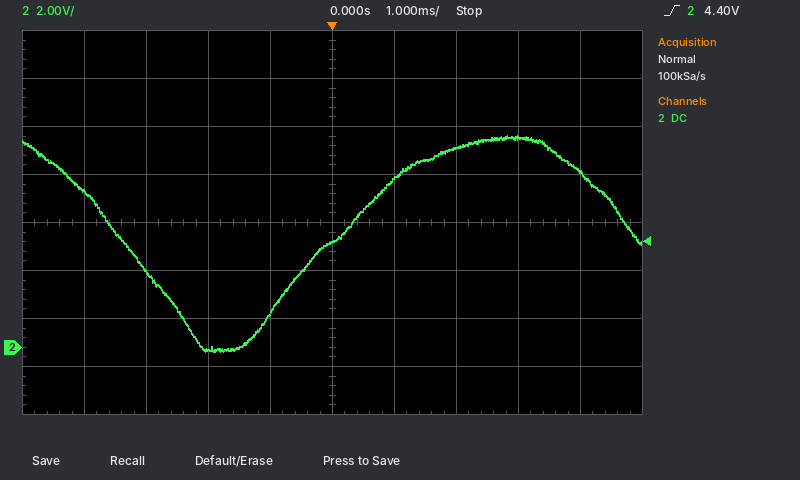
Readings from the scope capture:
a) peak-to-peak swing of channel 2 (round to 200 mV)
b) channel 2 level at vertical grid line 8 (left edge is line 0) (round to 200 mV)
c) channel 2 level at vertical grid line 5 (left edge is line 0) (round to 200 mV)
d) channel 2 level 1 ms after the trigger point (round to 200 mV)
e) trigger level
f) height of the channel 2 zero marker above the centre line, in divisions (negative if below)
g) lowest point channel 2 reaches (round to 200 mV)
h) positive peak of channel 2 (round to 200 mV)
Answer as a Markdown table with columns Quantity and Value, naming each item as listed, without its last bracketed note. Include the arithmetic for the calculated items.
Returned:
| Quantity | Value |
|---|---|
| peak-to-peak swing of channel 2 | 8.8 V − (-200 mV) = 9.0 V |
| channel 2 level at vertical grid line 8 (left edge is line 0) | 8.8 V |
| channel 2 level at vertical grid line 5 (left edge is line 0) | 4.4 V |
| channel 2 level 1 ms after the trigger point | 7.0 V |
| trigger level | 4.40 V |
| height of the channel 2 zero marker above the centre line, in divisions | -2.6 div |
| lowest point channel 2 reaches | -200 mV |
| positive peak of channel 2 | 8.8 V |
